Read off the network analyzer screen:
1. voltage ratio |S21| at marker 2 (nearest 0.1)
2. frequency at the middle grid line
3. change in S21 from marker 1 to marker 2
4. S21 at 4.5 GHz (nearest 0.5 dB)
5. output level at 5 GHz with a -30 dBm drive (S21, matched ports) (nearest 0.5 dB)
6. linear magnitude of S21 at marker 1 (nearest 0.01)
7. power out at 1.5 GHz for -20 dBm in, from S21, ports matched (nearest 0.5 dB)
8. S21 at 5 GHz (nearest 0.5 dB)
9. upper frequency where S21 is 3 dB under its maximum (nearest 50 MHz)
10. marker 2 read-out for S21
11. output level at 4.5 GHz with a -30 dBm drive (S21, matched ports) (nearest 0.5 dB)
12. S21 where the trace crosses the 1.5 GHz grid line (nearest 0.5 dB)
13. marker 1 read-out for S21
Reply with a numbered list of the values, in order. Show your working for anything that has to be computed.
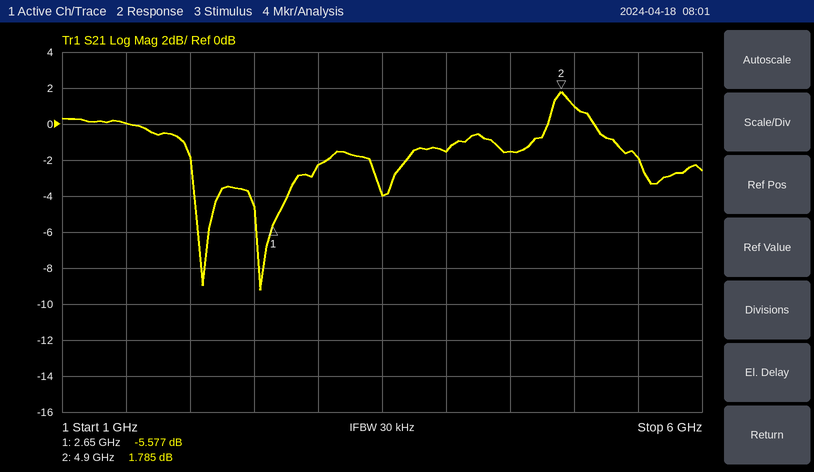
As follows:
1. 10^(1.785/20) ≈ 1.2
2. 3.5 GHz
3. 1.785 − (-5.577) = 7.362 dB
4. -1.5 dB
5. -30 dBm + (1.0 dB) = -29.0 dBm
6. 10^(-5.577/20) ≈ 0.53
7. -20 dBm + (0.0 dB) = -20.0 dBm
8. 1.0 dB
9. 5.35 GHz
10. 1.785 dB
11. -30 dBm + (-1.5 dB) = -31.5 dBm
12. 0.0 dB
13. -5.577 dB
